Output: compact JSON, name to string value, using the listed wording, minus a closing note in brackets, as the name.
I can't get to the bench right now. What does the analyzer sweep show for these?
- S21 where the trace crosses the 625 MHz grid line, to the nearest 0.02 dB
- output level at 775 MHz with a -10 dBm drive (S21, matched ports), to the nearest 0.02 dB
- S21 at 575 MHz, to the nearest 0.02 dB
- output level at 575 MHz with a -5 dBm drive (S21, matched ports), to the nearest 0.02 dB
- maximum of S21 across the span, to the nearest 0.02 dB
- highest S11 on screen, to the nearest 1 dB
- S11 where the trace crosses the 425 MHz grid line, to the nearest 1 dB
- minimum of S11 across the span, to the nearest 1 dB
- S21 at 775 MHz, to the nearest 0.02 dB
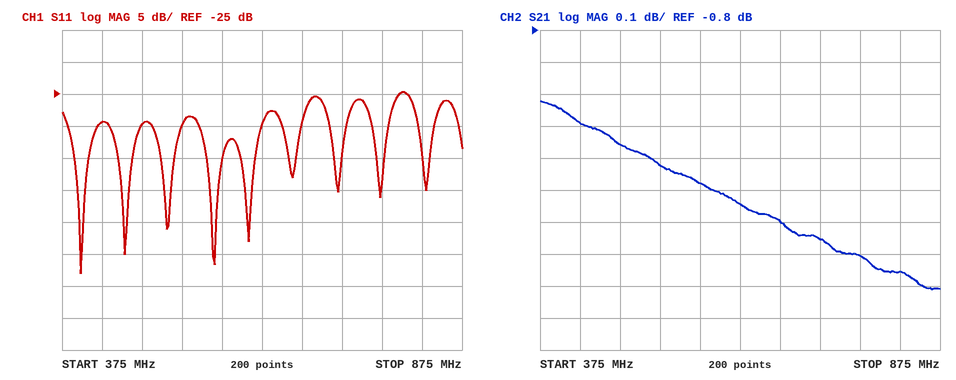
{"S21 where the trace crosses the 625 MHz grid line, to the nearest 0.02 dB": "-1.34 dB", "output level at 775 MHz with a -10 dBm drive (S21, matched ports), to the nearest 0.02 dB": "-11.50 dBm", "S21 at 575 MHz, to the nearest 0.02 dB": "-1.28 dB", "output level at 575 MHz with a -5 dBm drive (S21, matched ports), to the nearest 0.02 dB": "-6.28 dBm", "maximum of S21 across the span, to the nearest 0.02 dB": "-1.02 dB", "highest S11 on screen, to the nearest 1 dB": "-25 dB", "S11 where the trace crosses the 425 MHz grid line, to the nearest 1 dB": "-29 dB", "minimum of S11 across the span, to the nearest 1 dB": "-53 dB", "S21 at 775 MHz, to the nearest 0.02 dB": "-1.50 dB"}
